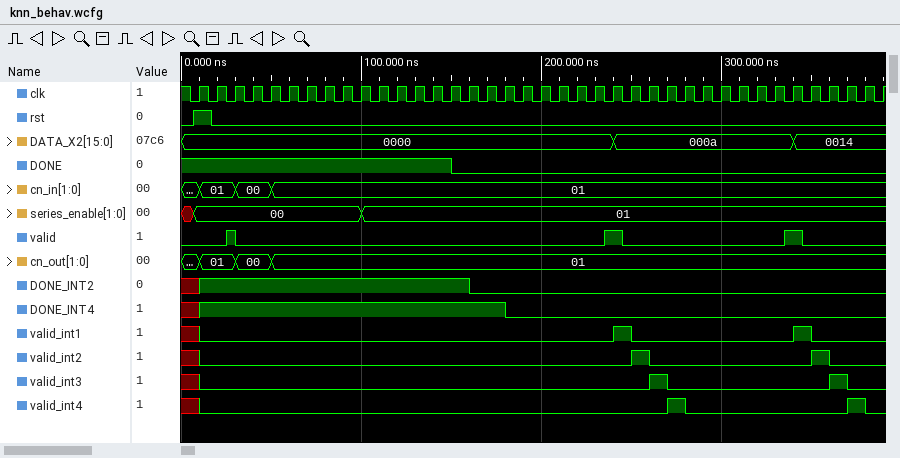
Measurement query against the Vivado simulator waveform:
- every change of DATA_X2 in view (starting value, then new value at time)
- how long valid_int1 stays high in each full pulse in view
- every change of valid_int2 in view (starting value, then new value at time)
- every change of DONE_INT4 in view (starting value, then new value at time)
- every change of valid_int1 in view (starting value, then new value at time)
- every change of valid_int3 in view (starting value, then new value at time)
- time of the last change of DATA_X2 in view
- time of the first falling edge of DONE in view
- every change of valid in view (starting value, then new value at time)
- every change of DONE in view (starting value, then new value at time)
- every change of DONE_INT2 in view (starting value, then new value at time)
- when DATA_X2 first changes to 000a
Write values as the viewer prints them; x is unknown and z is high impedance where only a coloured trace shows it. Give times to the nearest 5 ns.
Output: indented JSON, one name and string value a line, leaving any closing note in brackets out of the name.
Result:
{
  "every change of DATA_X2 in view": "0000, 000a at 240 ns, 0014 at 340 ns",
  "how long valid_int1 stays high in each full pulse in view": "10 ns, 10 ns",
  "every change of valid_int2 in view": "x, 0 at 10 ns, 1 at 250 ns, 0 at 260 ns, 1 at 350 ns, 0 at 360 ns",
  "every change of DONE_INT4 in view": "x, 1 at 10 ns, 0 at 180 ns",
  "every change of valid_int1 in view": "x, 0 at 10 ns, 1 at 240 ns, 0 at 250 ns, 1 at 340 ns, 0 at 350 ns",
  "every change of valid_int3 in view": "x, 0 at 10 ns, 1 at 260 ns, 0 at 270 ns, 1 at 360 ns, 0 at 370 ns",
  "time of the last change of DATA_X2 in view": "340 ns",
  "time of the first falling edge of DONE in view": "150 ns",
  "every change of valid in view": "0, 1 at 25 ns, 0 at 30 ns, 1 at 235 ns, 0 at 245 ns, 1 at 335 ns, 0 at 345 ns",
  "every change of DONE in view": "1, 0 at 150 ns",
  "every change of DONE_INT2 in view": "x, 1 at 10 ns, 0 at 160 ns",
  "when DATA_X2 first changes to 000a": "240 ns"
}
